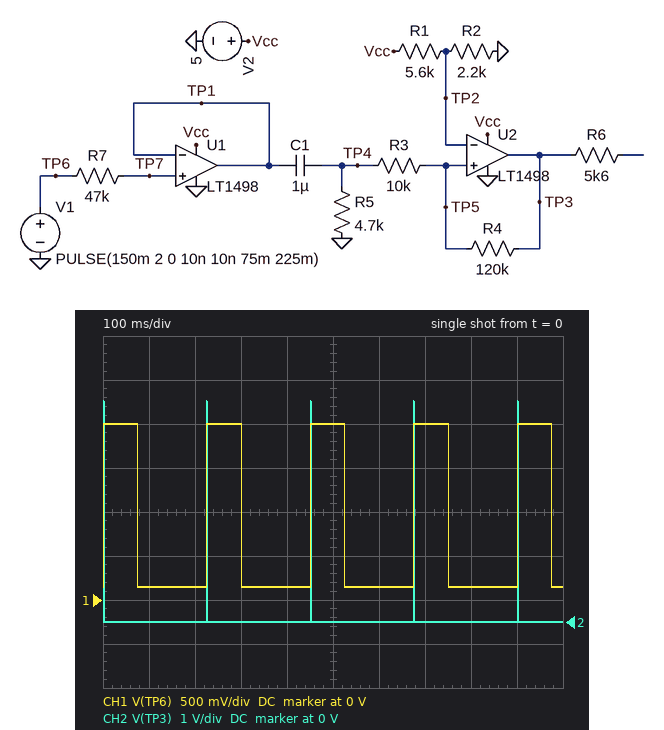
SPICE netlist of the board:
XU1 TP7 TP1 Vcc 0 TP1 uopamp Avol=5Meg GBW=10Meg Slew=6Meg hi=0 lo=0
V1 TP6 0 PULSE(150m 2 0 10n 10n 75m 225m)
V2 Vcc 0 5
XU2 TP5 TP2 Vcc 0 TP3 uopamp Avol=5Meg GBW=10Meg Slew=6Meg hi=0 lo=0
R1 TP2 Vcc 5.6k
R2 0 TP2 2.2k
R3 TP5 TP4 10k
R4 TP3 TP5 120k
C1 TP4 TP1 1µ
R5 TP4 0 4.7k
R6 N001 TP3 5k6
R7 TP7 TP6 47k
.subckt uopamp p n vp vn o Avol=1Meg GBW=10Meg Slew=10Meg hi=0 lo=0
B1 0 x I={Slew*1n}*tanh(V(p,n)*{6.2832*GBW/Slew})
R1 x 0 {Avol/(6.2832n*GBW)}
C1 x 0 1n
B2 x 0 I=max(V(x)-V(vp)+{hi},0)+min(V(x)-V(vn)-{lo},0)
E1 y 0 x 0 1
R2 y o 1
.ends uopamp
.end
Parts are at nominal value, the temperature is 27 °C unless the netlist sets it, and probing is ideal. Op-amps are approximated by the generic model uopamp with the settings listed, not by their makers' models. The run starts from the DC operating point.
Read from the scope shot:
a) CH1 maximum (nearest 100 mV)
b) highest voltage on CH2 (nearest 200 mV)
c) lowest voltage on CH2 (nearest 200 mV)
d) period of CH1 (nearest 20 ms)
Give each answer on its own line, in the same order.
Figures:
2.0 V
5.0 V
0 V
220 ms
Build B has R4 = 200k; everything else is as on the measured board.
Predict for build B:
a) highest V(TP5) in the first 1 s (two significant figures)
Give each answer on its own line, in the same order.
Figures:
2.0 V
